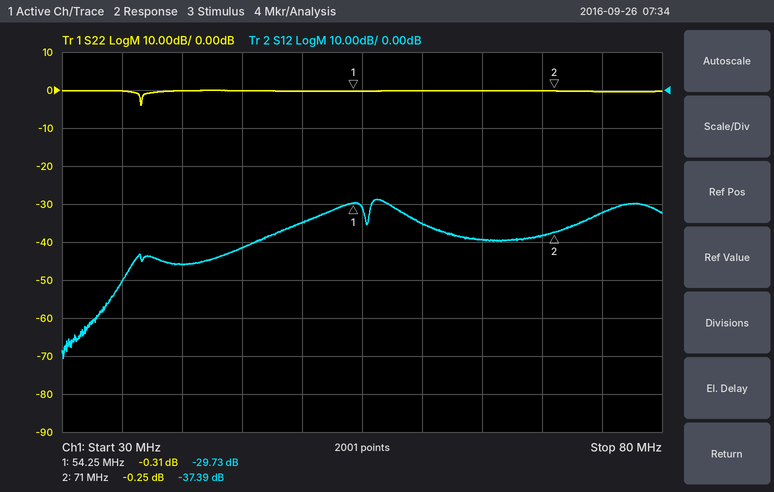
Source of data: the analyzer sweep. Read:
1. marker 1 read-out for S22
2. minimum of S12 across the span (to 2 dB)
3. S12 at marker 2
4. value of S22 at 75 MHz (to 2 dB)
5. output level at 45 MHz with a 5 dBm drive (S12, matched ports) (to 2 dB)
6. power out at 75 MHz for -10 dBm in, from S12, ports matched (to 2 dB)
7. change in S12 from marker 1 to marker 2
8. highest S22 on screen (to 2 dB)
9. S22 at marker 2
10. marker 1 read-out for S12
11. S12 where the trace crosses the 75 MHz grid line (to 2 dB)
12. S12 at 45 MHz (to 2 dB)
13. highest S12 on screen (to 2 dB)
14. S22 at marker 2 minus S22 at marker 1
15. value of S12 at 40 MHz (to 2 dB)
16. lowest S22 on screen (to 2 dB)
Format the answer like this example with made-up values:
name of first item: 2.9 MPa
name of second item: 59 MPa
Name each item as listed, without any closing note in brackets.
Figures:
marker 1 read-out for S22: -0.31 dB
minimum of S12 across the span: -70 dB
S12 at marker 2: -37.39 dB
value of S22 at 75 MHz: 0 dB
output level at 45 MHz with a 5 dBm drive (S12, matched ports): -36 dBm
power out at 75 MHz for -10 dBm in, from S12, ports matched: -42 dBm
change in S12 from marker 1 to marker 2: -7.66 dB
highest S22 on screen: 0 dB
S22 at marker 2: -0.25 dB
marker 1 read-out for S12: -29.73 dB
S12 where the trace crosses the 75 MHz grid line: -32 dB
S12 at 45 MHz: -42 dB
highest S12 on screen: -28 dB
S22 at marker 2 minus S22 at marker 1: 0.06 dB
value of S12 at 40 MHz: -46 dB
lowest S22 on screen: -4 dB
